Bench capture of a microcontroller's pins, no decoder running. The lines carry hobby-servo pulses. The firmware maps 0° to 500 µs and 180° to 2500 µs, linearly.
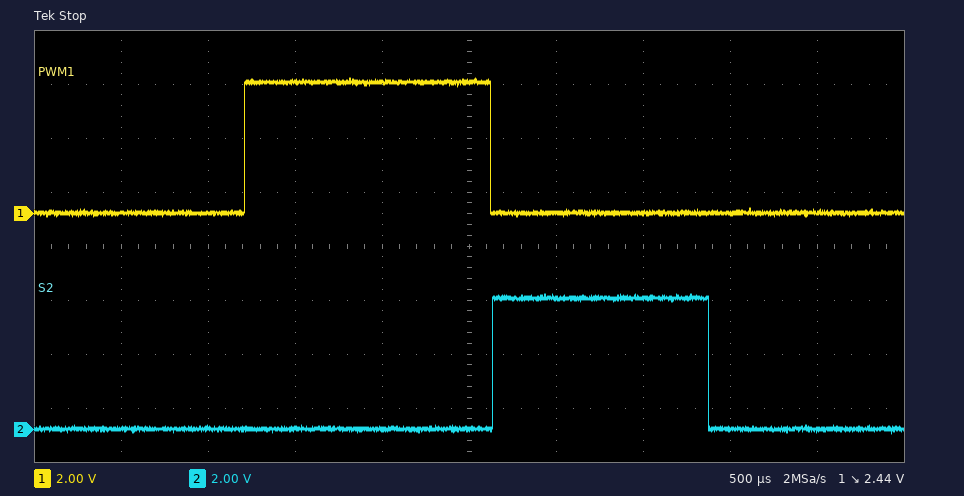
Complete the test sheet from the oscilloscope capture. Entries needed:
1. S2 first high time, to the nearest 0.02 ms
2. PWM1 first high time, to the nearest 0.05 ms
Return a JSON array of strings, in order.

["1.24 ms", "1.40 ms"]
